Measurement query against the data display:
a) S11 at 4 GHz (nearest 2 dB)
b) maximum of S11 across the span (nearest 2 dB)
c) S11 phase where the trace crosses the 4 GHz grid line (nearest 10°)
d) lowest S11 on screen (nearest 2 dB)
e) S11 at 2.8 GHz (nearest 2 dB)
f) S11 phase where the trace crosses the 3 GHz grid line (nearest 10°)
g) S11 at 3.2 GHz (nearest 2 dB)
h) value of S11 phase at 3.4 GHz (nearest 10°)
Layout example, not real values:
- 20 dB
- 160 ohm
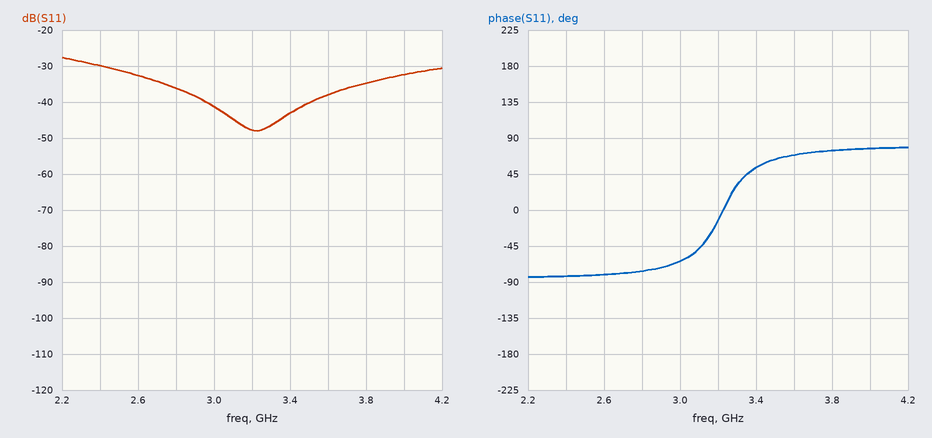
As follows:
- -32 dB
- -28 dB
- 80°
- -48 dB
- -36 dB
- -60°
- -48 dB
- 50°
